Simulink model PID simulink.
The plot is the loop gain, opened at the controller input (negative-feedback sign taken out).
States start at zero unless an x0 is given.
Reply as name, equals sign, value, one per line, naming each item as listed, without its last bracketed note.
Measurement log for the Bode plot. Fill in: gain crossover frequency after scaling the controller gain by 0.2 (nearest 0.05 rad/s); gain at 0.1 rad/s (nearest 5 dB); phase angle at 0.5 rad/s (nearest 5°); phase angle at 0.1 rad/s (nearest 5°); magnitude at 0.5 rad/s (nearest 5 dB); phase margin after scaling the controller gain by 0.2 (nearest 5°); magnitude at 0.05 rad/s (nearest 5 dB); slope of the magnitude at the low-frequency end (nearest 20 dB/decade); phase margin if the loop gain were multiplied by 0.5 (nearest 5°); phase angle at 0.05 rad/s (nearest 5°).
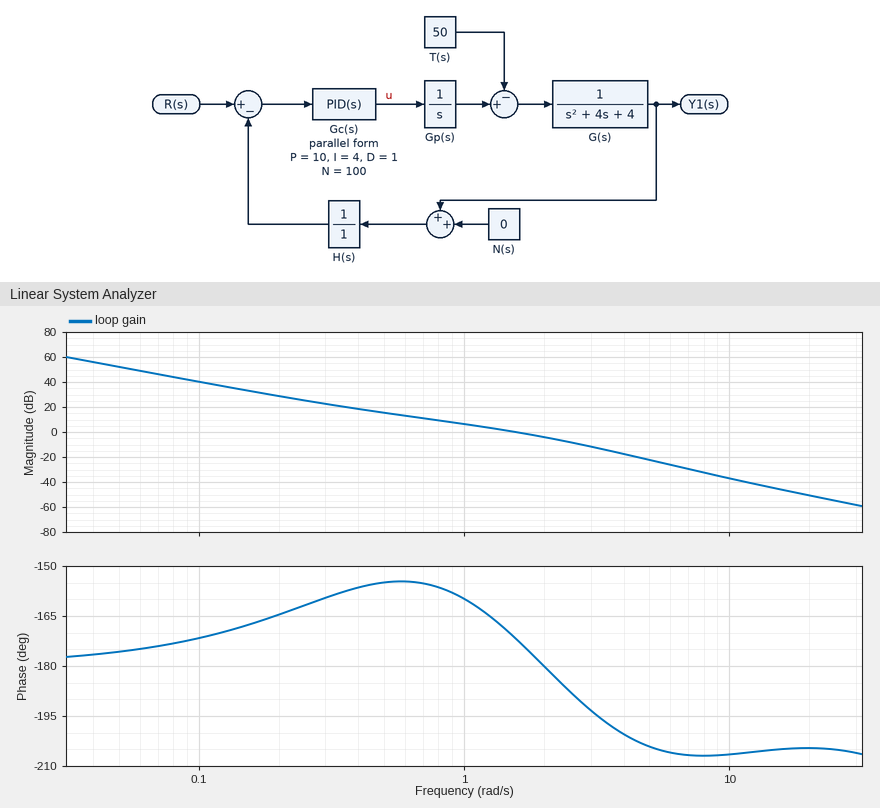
gain crossover frequency after scaling the controller gain by 0.2 = 0.55 rad/s
gain at 0.1 rad/s = 40 dB
phase angle at 0.5 rad/s = -155°
phase angle at 0.1 rad/s = -170°
magnitude at 0.5 rad/s = 15 dB
phase margin after scaling the controller gain by 0.2 = 25°
magnitude at 0.05 rad/s = 50 dB
slope of the magnitude at the low-frequency end = -40 dB/decade
phase margin if the loop gain were multiplied by 0.5 = 20°
phase angle at 0.05 rad/s = -175°
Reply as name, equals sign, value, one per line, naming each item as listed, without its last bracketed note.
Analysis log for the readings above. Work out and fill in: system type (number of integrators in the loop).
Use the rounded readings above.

system type = 2
